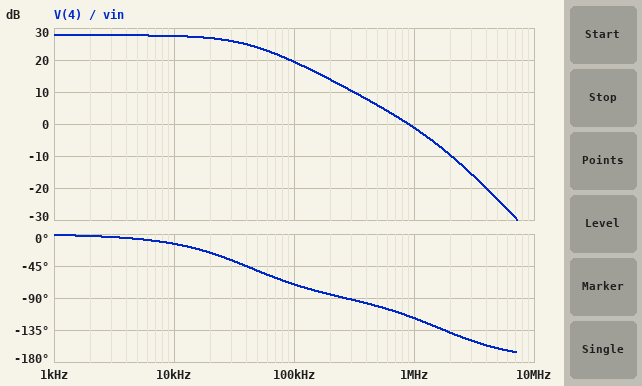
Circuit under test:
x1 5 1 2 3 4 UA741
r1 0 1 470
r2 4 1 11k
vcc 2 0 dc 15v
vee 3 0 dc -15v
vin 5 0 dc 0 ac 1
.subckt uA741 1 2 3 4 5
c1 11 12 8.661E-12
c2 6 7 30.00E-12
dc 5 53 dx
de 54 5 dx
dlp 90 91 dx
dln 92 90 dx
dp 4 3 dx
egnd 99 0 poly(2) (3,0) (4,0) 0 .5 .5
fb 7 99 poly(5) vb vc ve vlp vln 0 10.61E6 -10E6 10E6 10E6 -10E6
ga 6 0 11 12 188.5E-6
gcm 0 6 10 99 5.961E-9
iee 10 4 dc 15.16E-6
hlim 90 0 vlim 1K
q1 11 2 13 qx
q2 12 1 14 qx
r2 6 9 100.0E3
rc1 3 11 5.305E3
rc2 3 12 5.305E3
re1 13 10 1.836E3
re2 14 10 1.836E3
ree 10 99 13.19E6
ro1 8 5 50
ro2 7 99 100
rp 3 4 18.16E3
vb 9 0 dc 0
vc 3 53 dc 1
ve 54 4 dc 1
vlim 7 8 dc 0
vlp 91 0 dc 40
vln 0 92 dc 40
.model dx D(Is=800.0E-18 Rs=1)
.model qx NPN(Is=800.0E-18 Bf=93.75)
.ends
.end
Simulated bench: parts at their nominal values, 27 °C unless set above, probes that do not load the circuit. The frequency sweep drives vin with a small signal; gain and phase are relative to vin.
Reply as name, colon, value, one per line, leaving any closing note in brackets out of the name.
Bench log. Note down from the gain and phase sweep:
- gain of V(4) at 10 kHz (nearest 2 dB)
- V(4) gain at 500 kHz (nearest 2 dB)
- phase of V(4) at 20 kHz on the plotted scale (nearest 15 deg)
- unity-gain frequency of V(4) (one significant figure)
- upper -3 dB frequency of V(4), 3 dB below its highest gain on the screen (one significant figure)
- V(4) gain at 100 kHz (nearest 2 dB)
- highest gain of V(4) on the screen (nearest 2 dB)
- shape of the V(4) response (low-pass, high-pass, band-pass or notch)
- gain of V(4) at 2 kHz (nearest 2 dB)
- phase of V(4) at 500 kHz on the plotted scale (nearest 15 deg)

gain of V(4) at 10 kHz: 28 dB
V(4) gain at 500 kHz: 6 dB
phase of V(4) at 20 kHz on the plotted scale: -30 deg
unity-gain frequency of V(4): 900 kHz
upper -3 dB frequency of V(4), 3 dB below its highest gain on the screen: 40 kHz
V(4) gain at 100 kHz: 20 dB
highest gain of V(4) on the screen: 28 dB
shape of the V(4) response: low-pass
gain of V(4) at 2 kHz: 28 dB
phase of V(4) at 500 kHz on the plotted scale: -105 deg
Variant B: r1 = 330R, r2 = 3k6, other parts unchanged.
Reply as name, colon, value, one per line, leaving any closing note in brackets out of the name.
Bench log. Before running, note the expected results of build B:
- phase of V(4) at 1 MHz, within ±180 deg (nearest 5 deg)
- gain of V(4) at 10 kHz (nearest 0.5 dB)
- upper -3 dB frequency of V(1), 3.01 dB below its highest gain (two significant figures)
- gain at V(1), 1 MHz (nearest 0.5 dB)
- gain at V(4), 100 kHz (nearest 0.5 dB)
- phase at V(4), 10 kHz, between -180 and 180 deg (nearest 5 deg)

phase of V(4) at 1 MHz, within ±180 deg: -115 deg
gain of V(4) at 10 kHz: 21.5 dB
upper -3 dB frequency of V(1), 3.01 dB below its highest gain: 87 kHz
gain at V(1), 1 MHz: -22.5 dB
gain at V(4), 100 kHz: 18.0 dB
phase at V(4), 10 kHz, between -180 and 180 deg: -5 deg
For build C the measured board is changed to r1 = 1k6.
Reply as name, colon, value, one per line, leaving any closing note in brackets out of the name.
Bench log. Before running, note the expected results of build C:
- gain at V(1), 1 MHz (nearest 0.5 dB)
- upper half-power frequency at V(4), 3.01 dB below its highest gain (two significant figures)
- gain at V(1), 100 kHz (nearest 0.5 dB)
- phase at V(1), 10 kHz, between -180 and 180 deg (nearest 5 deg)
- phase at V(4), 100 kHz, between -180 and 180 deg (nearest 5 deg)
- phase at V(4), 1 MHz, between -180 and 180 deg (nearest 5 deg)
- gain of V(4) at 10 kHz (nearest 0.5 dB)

gain at V(1), 1 MHz: -19.0 dB
upper half-power frequency at V(4), 3.01 dB below its highest gain: 140 kHz
gain at V(1), 100 kHz: -2.0 dB
phase at V(1), 10 kHz, between -180 and 180 deg: -5 deg
phase at V(4), 100 kHz, between -180 and 180 deg: -40 deg
phase at V(4), 1 MHz, between -180 and 180 deg: -115 deg
gain of V(4) at 10 kHz: 18.0 dB
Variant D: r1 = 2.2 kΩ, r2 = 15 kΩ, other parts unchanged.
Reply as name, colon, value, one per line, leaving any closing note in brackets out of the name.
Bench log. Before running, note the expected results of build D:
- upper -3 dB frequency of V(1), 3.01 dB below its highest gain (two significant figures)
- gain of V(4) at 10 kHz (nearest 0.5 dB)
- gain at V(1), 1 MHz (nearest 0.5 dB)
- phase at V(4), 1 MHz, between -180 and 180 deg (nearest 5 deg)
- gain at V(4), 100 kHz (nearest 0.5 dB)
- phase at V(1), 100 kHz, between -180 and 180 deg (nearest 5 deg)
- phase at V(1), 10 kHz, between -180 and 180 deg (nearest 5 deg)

upper -3 dB frequency of V(1), 3.01 dB below its highest gain: 140 kHz
gain of V(4) at 10 kHz: 18.0 dB
gain at V(1), 1 MHz: -19.0 dB
phase at V(4), 1 MHz, between -180 and 180 deg: -115 deg
gain at V(4), 100 kHz: 16.0 dB
phase at V(1), 100 kHz, between -180 and 180 deg: -40 deg
phase at V(1), 10 kHz, between -180 and 180 deg: -5 deg
